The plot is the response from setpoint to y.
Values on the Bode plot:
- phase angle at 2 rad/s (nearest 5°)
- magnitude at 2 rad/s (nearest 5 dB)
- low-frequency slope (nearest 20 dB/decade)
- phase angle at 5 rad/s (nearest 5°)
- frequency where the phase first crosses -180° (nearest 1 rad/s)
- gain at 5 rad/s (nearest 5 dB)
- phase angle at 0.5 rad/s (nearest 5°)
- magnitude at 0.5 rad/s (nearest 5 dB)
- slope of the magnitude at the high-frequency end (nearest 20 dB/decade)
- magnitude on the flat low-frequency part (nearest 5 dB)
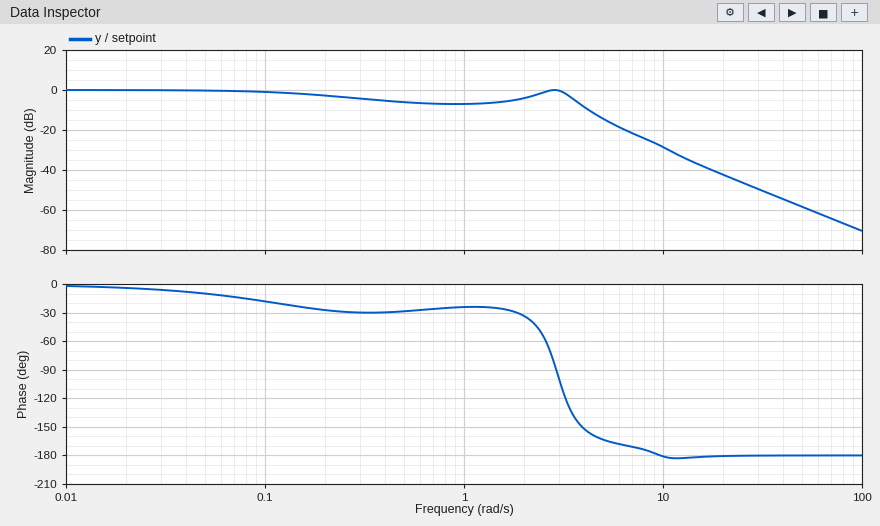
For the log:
-35°
-5 dB
0 dB/decade
-165°
10 rad/s
-15 dB
-30°
-5 dB
-40 dB/decade
0 dB
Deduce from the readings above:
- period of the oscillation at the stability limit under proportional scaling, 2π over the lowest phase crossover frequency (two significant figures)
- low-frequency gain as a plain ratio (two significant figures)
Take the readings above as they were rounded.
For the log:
0.63 s
1.0
